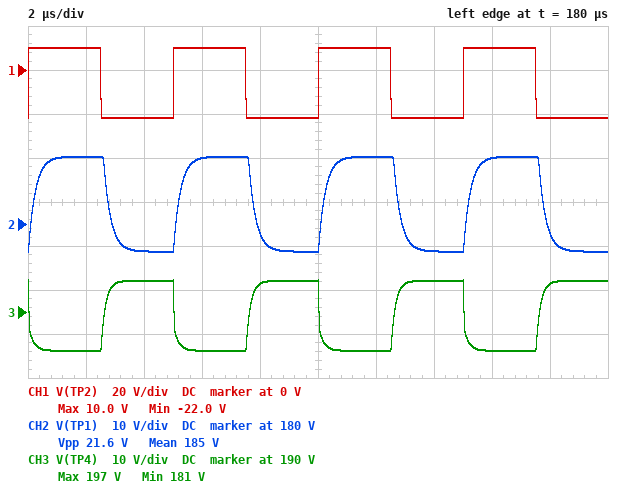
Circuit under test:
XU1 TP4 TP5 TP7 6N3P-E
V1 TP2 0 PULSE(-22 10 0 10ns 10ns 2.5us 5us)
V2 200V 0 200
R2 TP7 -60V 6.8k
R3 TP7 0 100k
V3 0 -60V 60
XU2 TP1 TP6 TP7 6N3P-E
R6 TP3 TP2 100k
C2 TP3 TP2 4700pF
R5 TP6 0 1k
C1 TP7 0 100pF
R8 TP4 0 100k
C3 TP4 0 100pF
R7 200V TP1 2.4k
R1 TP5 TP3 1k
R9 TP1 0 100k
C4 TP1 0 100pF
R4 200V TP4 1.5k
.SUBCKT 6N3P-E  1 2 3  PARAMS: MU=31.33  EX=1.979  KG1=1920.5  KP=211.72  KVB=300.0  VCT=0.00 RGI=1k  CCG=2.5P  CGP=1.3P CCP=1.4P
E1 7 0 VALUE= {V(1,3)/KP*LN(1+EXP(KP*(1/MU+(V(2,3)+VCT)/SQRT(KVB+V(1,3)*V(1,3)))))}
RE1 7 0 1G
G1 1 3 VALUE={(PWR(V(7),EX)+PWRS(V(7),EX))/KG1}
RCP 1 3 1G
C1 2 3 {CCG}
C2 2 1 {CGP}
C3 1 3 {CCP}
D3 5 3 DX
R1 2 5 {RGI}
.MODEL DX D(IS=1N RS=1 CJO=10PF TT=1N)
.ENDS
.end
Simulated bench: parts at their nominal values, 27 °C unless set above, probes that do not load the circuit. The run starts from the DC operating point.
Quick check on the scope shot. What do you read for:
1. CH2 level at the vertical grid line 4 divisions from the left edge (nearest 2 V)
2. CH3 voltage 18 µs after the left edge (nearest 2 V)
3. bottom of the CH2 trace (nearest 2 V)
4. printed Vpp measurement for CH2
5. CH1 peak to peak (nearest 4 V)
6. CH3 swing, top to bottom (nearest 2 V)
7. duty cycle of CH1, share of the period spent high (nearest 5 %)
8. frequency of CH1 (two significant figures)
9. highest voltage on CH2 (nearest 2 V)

178 V
196 V
174 V
21.6 V
32 V
16 V
50 %
200 kHz
196 V
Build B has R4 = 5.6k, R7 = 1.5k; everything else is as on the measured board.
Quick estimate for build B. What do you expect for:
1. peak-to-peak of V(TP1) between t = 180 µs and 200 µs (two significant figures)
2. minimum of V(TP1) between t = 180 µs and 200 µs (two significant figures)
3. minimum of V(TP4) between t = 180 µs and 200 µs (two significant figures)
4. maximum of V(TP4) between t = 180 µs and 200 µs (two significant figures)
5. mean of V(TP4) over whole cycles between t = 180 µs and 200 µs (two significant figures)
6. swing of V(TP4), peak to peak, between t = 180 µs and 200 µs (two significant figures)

14 V
180 V
130 V
190 V
160 V
55 V
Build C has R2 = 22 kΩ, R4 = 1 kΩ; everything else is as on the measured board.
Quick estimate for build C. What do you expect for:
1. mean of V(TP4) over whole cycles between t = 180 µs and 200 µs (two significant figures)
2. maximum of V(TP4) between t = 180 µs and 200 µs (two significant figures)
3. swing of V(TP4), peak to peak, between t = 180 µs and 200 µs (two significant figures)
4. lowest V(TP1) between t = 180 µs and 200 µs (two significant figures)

200 V
200 V
7.5 V
190 V
